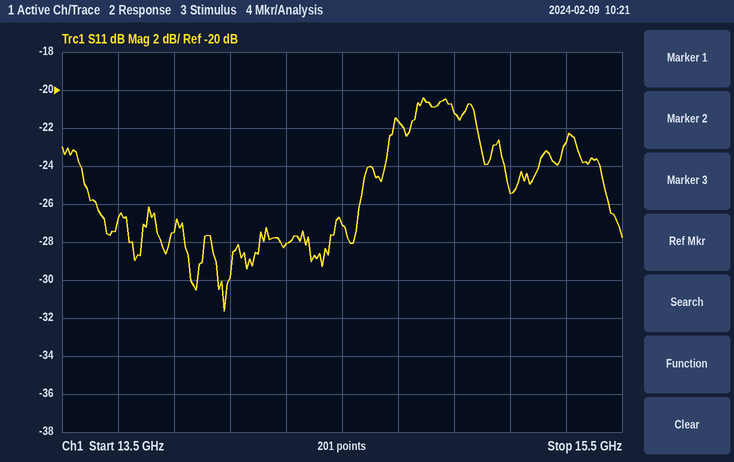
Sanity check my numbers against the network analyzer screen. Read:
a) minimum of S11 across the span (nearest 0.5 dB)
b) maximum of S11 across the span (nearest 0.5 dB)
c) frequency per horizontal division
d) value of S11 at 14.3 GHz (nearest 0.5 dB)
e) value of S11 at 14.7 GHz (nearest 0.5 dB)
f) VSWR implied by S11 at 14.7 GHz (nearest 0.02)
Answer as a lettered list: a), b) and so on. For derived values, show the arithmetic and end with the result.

a) -31.5 dB
b) -20.5 dB
c) 200 MHz
d) -28.0 dB
e) -21.5 dB
f) |Γ| = 10^(-21.5/20) = 0.0841; VSWR = (1 + 0.0841)/(1 − 0.0841) ≈ 1.18
